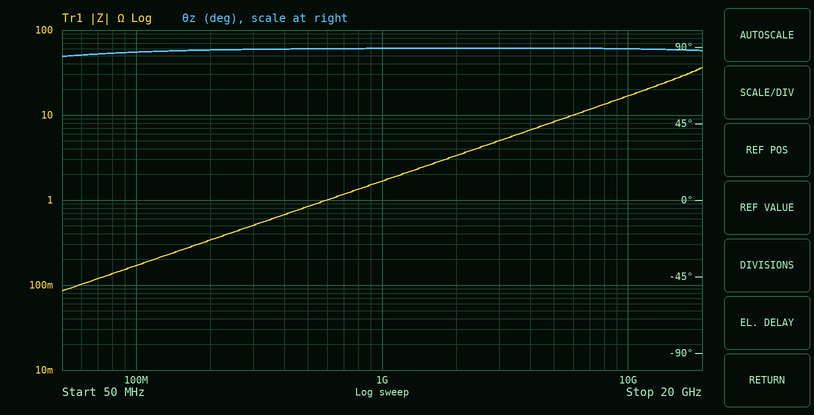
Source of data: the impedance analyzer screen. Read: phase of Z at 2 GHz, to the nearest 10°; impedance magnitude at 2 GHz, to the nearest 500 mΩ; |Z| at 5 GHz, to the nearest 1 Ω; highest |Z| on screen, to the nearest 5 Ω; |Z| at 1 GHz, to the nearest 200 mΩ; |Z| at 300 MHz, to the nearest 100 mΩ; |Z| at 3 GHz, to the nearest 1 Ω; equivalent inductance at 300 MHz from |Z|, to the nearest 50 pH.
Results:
90°
3.5 Ω
8 Ω
35 Ω
1.6 Ω
500 mΩ
5 Ω
250 pH
